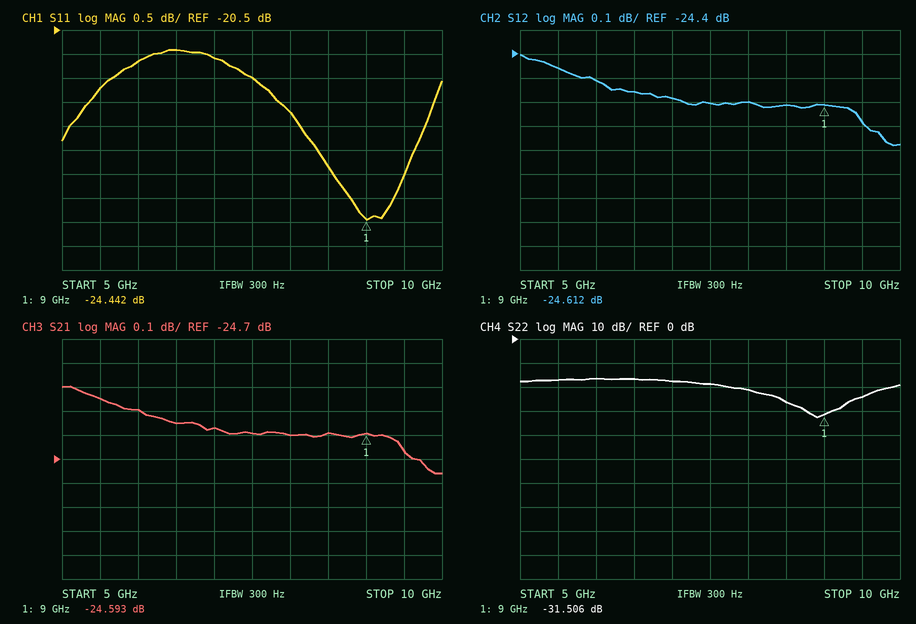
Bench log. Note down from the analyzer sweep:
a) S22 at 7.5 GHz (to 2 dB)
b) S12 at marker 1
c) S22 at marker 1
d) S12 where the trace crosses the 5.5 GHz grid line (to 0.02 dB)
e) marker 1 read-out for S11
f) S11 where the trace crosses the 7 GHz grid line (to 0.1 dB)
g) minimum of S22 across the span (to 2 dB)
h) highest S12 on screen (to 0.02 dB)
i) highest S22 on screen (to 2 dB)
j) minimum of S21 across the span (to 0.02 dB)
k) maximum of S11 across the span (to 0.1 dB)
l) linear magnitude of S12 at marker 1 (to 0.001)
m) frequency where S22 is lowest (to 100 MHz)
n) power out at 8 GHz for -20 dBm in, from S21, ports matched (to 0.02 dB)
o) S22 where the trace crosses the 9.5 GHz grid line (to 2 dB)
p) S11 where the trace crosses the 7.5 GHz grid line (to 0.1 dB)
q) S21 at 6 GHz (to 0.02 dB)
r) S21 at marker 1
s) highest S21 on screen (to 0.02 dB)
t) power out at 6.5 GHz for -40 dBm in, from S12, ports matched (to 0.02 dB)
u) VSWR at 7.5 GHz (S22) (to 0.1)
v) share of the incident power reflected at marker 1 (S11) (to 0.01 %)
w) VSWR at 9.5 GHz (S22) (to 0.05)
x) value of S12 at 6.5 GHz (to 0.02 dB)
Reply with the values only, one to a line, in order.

-18 dB
-24.612 dB
-31.506 dB
-24.46 dB
-24.442 dB
-21.1 dB
-32 dB
-24.40 dB
-16 dB
-24.76 dB
-20.9 dB
0.059
8.9 GHz
-44.60 dBm
-24 dB
-21.5 dB
-24.50 dB
-24.593 dB
-24.40 dB
-64.56 dBm
1.3
0.36 %
1.15
-24.56 dB
